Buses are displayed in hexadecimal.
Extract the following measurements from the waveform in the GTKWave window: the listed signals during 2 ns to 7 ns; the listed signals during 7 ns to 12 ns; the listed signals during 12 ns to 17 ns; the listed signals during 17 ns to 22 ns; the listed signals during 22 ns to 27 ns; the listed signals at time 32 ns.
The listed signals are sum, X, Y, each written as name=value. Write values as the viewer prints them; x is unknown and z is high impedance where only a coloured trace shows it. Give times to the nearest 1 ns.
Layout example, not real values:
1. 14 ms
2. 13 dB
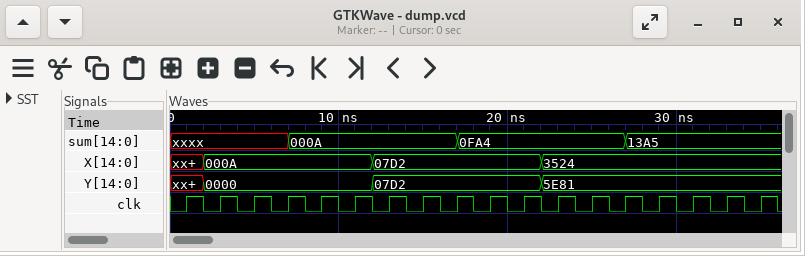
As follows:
1. sum=xxxx, X=000A, Y=0000
2. sum=000A, X=000A, Y=0000
3. sum=000A, X=07D2, Y=07D2
4. sum=0FA4, X=07D2, Y=07D2
5. sum=0FA4, X=3524, Y=5E81
6. sum=13A5, X=3524, Y=5E81
